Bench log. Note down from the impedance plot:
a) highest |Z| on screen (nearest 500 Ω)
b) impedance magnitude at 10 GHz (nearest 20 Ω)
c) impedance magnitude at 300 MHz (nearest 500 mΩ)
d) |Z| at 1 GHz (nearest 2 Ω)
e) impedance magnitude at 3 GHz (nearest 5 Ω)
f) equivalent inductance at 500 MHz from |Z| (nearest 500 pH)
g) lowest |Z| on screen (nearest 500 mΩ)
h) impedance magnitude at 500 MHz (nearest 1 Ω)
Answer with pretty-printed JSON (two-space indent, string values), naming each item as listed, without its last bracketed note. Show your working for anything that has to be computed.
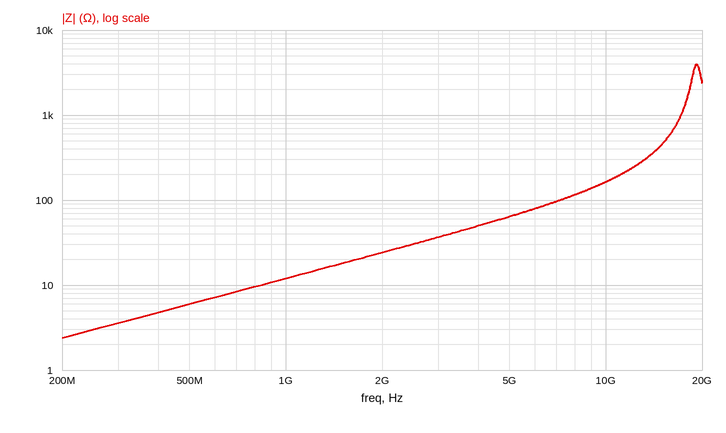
{
  "highest |Z| on screen": "4.0 kΩ",
  "impedance magnitude at 10 GHz": "160 Ω",
  "impedance magnitude at 300 MHz": "3.5 Ω",
  "|Z| at 1 GHz": "12 Ω",
  "impedance magnitude at 3 GHz": "35 Ω",
  "equivalent inductance at 500 MHz from |Z|": "L = 6 Ω/(2π × 500 MHz) ≈ 1.91 nH, so 2.0 nH to the nearest 500 pH",
  "lowest |Z| on screen": "2.5 Ω",
  "impedance magnitude at 500 MHz": "6 Ω"
}
